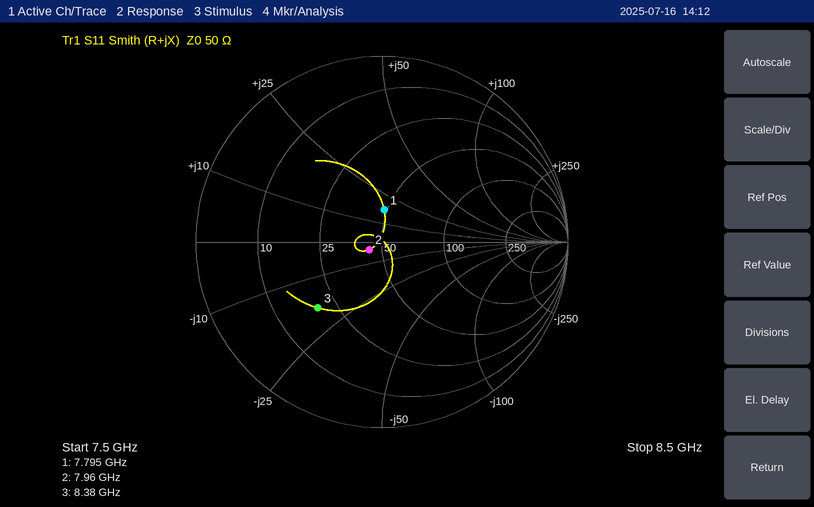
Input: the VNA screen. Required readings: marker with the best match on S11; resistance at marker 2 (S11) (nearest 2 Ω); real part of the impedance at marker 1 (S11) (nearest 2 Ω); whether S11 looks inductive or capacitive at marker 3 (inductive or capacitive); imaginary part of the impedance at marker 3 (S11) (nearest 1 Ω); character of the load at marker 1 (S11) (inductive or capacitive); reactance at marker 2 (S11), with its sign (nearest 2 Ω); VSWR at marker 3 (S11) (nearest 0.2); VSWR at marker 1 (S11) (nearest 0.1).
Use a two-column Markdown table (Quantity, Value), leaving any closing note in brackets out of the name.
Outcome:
| Quantity | Value |
|---|---|
| marker with the best match on S11 | marker 2 |
| resistance at marker 2 (S11) | 44 Ω |
| real part of the impedance at marker 1 (S11) | 48 Ω |
| whether S11 looks inductive or capacitive at marker 3 | capacitive |
| imaginary part of the impedance at marker 3 (S11) | -18 Ω |
| character of the load at marker 1 (S11) | inductive |
| reactance at marker 2 (S11), with its sign | -4 Ω |
| VSWR at marker 3 (S11) | 3.0 |
| VSWR at marker 1 (S11) | 1.4 |
